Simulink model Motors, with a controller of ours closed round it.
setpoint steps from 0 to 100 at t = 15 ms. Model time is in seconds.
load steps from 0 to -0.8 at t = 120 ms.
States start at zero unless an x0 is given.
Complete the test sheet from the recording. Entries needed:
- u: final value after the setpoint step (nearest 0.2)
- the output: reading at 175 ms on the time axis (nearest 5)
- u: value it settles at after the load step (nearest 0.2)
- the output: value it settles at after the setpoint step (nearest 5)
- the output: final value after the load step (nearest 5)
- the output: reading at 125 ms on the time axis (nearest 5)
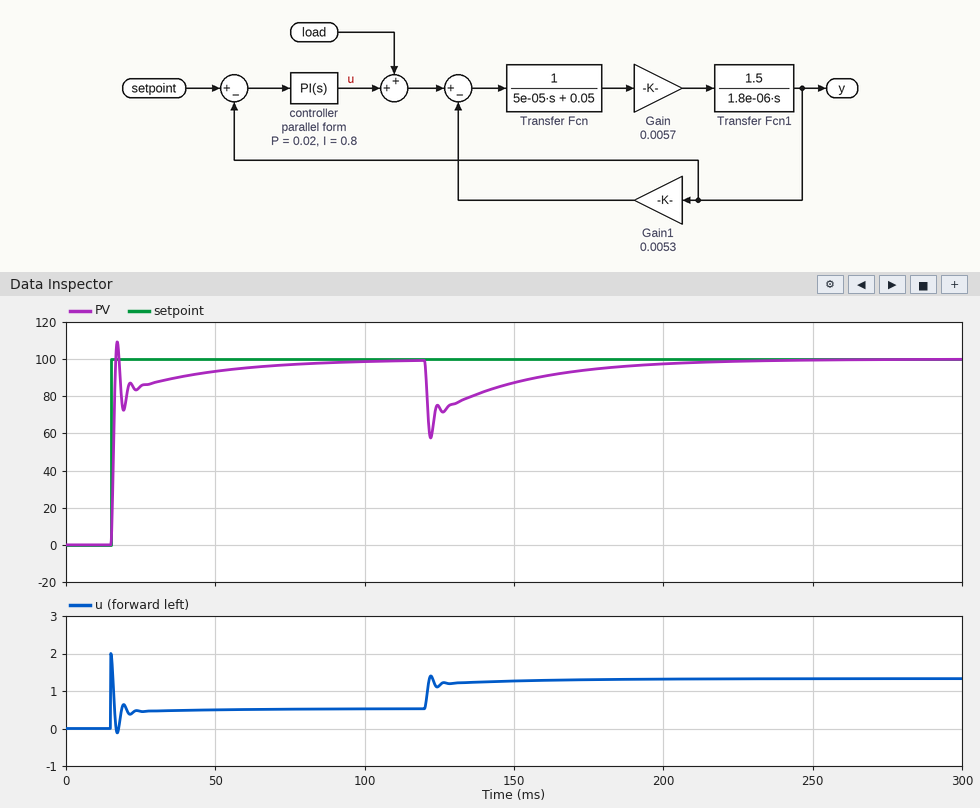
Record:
0.6
95
1.4
100
100
75
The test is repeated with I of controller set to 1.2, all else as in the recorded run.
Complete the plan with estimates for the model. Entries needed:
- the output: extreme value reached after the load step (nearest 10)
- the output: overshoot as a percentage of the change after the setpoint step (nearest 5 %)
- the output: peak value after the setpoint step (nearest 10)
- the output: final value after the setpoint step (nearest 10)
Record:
60
10 %
110
100
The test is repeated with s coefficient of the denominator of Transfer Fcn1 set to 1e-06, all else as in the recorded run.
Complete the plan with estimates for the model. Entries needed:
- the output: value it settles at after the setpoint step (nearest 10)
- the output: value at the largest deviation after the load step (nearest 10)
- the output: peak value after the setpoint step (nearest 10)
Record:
100
50
120
